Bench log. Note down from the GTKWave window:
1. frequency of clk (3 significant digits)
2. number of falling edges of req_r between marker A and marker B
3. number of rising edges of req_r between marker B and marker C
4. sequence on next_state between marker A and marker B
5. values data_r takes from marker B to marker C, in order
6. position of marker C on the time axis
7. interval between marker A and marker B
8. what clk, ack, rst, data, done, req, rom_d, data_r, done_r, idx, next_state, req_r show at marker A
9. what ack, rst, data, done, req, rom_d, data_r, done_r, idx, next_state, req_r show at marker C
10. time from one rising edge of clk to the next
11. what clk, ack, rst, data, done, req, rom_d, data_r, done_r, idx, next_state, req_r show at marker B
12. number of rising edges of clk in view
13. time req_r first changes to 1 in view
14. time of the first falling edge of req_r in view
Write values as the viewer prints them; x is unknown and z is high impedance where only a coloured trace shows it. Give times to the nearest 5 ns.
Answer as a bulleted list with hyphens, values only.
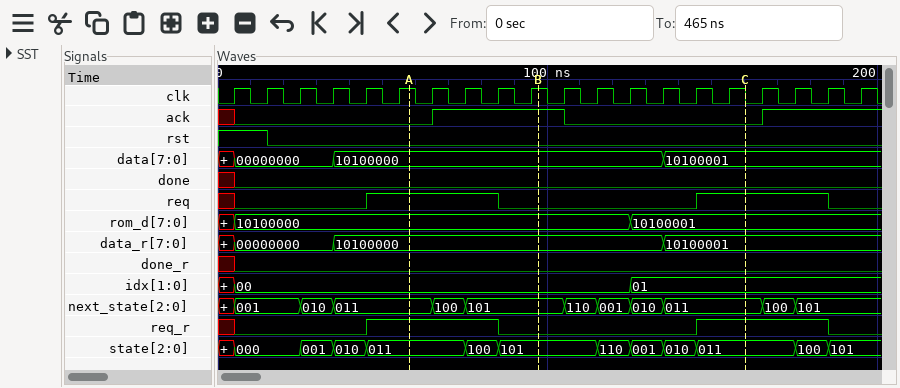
- 100 MHz
- 1
- 1
- 011, 100, 101
- 10100000, 10100001
- 160 ns
- 40 ns
- clk=1, ack=0, rst=0, data=10100000, done=0, req=1, rom_d=10100000, data_r=10100000, done_r=0, idx=00, next_state=011, req_r=1
- ack=0, rst=0, data=10100001, done=0, req=1, rom_d=10100001, data_r=10100001, done_r=0, idx=01, next_state=011, req_r=1
- 10 ns
- clk=1, ack=1, rst=0, data=10100000, done=0, req=0, rom_d=10100000, data_r=10100000, done_r=0, idx=00, next_state=101, req_r=0
- 20
- 45 ns
- 85 ns
